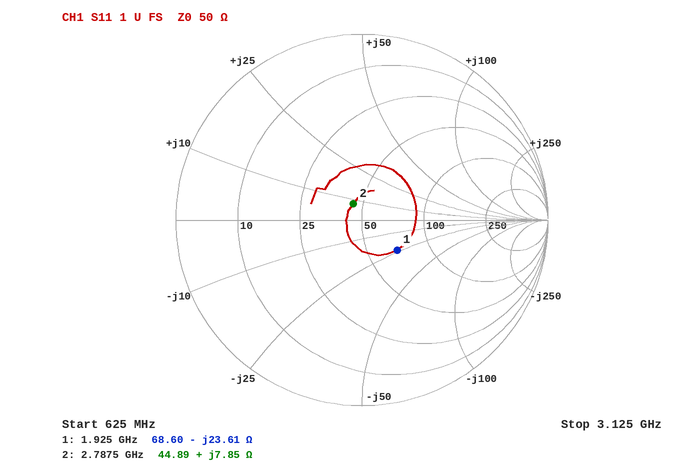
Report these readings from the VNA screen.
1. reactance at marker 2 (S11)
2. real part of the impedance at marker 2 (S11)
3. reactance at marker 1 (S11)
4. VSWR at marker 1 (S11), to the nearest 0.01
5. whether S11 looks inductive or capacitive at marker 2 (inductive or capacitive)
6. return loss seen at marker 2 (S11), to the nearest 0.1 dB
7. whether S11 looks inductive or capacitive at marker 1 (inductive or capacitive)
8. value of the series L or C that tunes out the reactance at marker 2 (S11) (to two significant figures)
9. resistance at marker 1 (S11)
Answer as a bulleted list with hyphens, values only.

- +7.85 Ω
- 44.89 Ω
- -23.61 Ω
- 1.66
- inductive
- 20.1 dB
- capacitive
- 7.3 pF
- 68.60 Ω
